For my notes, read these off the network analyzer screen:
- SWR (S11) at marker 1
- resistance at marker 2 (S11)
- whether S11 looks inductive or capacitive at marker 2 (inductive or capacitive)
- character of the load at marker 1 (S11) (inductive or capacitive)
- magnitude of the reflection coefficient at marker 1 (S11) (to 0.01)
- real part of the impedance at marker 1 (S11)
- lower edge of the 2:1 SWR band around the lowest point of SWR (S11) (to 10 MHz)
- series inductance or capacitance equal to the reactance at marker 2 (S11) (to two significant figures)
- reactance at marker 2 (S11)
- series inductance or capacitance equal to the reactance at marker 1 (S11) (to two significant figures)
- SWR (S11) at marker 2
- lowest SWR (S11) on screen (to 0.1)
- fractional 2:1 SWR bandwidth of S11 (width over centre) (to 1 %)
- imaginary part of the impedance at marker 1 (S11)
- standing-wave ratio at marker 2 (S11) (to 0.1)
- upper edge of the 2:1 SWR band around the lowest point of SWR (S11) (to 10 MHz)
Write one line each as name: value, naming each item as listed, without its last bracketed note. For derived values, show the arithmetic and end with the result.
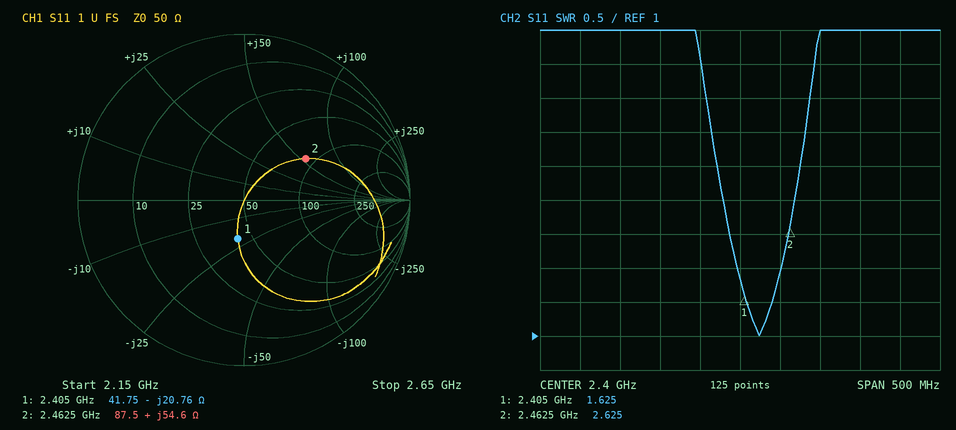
SWR (S11) at marker 1: 1.625
resistance at marker 2: 87.5 Ω
whether S11 looks inductive or capacitive at marker 2: inductive
character of the load at marker 1 (S11): capacitive
magnitude of the reflection coefficient at marker 1 (S11): 0.24
real part of the impedance at marker 1: 41.75 Ω
lower edge of the 2:1 SWR band around the lowest point of SWR (S11): 2.40 GHz
series inductance or capacitance equal to the reactance at marker 2 (S11): L = 54.6 Ω/(2π × 2.4625 GHz) ≈ 3.5 nH
reactance at marker 2: +54.6 Ω
series inductance or capacitance equal to the reactance at marker 1 (S11): C = 1/(2π × 2.405 GHz × 20.76 Ω) ≈ 3.2 pF
SWR (S11) at marker 2: 2.625
lowest SWR (S11) on screen: 1.0
fractional 2:1 SWR bandwidth of S11 (width over centre): 50 MHz / 2.425 GHz ≈ 2 %
imaginary part of the impedance at marker 1: -20.76 Ω
standing-wave ratio at marker 2 (S11): 2.6
upper edge of the 2:1 SWR band around the lowest point of SWR (S11): 2.45 GHz
